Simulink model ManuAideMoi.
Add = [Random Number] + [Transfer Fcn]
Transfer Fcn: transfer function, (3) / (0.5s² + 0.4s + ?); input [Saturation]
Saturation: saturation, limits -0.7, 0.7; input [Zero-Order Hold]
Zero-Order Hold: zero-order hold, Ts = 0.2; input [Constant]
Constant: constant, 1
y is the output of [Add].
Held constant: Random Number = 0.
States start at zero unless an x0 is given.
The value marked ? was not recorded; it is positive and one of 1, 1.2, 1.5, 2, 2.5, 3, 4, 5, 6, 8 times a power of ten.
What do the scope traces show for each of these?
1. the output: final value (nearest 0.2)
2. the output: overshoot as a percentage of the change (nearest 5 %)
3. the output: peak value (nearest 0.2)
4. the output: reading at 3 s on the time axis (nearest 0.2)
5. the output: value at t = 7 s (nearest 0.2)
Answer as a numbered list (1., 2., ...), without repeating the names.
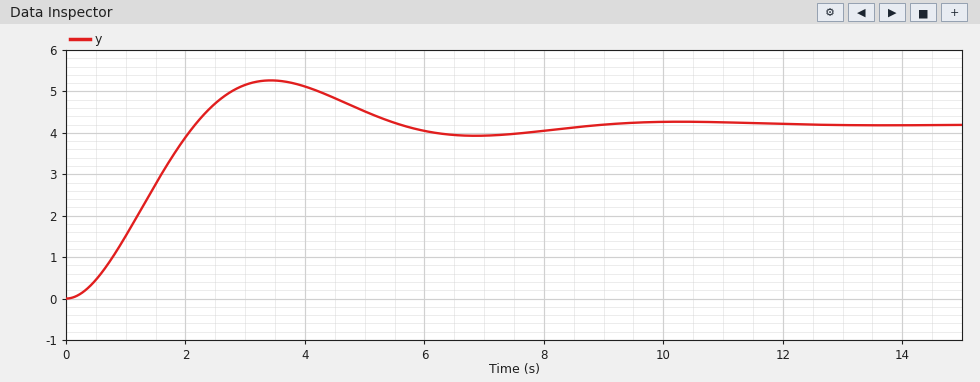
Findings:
1. 4.2
2. 25 %
3. 5.2
4. 5.2
5. 4.0
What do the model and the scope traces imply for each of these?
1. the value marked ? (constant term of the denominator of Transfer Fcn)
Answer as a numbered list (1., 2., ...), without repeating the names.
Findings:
1. 0.5
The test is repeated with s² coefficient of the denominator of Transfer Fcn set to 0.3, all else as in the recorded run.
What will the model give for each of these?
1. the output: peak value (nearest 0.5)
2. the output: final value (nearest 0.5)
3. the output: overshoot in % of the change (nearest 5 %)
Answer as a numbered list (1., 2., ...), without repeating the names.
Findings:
1. 5.0
2. 4.0
3. 15 %
